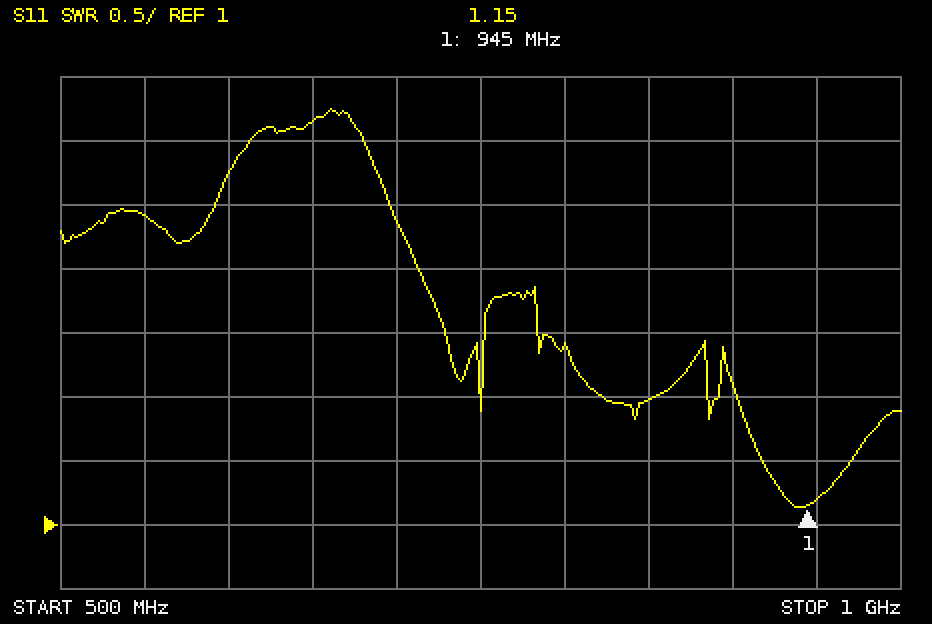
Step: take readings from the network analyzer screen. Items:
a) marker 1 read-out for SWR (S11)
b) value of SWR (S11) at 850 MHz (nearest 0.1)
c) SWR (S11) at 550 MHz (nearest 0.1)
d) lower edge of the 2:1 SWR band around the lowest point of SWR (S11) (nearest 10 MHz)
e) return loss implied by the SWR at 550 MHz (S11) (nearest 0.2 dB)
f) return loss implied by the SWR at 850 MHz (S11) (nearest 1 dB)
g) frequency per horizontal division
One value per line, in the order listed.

1.15
2.0
3.4
900 MHz
5.2 dB
10 dB
50 MHz
